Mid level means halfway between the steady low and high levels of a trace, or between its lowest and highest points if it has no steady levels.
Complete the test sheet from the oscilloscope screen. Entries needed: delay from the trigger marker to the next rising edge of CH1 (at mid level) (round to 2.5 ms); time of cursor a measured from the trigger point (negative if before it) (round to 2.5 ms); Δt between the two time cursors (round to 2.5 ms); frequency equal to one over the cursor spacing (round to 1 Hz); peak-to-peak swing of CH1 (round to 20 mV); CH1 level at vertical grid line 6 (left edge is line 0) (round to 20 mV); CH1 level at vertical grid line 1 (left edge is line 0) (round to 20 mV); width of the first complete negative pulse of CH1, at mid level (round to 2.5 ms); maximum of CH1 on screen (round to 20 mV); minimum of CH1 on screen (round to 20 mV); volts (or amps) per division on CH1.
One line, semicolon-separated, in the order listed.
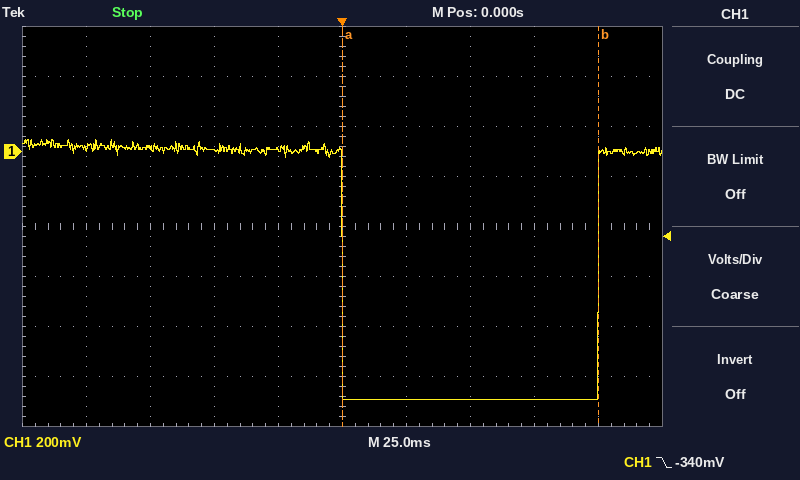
100.0 ms; 0.0 ms; 100.0 ms; 10 Hz; 1.04 V; -1.00 V; 20 mV; 100.0 ms; 40 mV; -1.00 V; 200 mV
